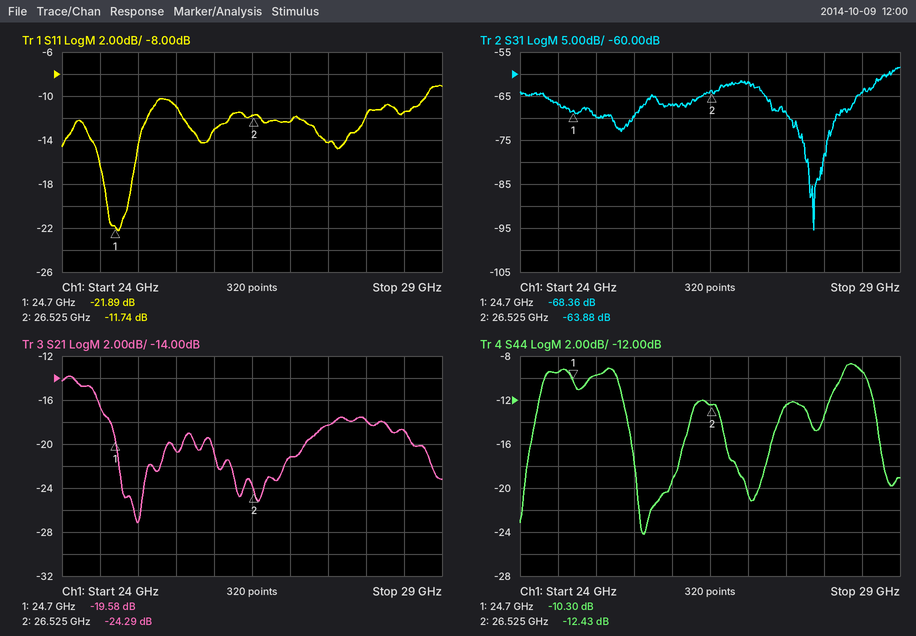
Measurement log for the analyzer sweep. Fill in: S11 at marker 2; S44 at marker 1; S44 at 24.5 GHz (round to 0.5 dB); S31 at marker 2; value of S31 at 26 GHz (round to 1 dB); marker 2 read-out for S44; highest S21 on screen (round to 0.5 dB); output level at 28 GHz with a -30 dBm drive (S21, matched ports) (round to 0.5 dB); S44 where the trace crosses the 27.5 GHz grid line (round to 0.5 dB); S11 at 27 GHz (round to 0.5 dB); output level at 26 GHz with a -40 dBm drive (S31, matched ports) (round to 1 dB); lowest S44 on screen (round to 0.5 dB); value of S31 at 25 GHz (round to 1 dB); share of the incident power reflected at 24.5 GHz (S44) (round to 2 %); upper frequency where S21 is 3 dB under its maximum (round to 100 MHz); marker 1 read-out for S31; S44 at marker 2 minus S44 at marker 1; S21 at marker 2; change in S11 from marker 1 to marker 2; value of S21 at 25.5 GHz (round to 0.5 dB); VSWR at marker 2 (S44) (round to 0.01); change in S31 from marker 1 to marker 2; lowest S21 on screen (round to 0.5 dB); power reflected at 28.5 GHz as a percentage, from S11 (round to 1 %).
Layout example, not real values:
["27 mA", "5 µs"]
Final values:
["-11.74 dB", "-10.30 dB", "-9.5 dB", "-63.88 dB", "-67 dB", "-12.43 dB", "-14.0 dB", "-48.0 dBm", "-12.5 dB", "-12.5 dB", "-107 dBm", "-24.0 dB", "-70 dB", "12 %", "24.5 GHz", "-68.36 dB", "-2.13 dB", "-24.29 dB", "10.15 dB", "-20.5 dB", "1.63", "4.48 dB", "-27.0 dB", "7 %"]
